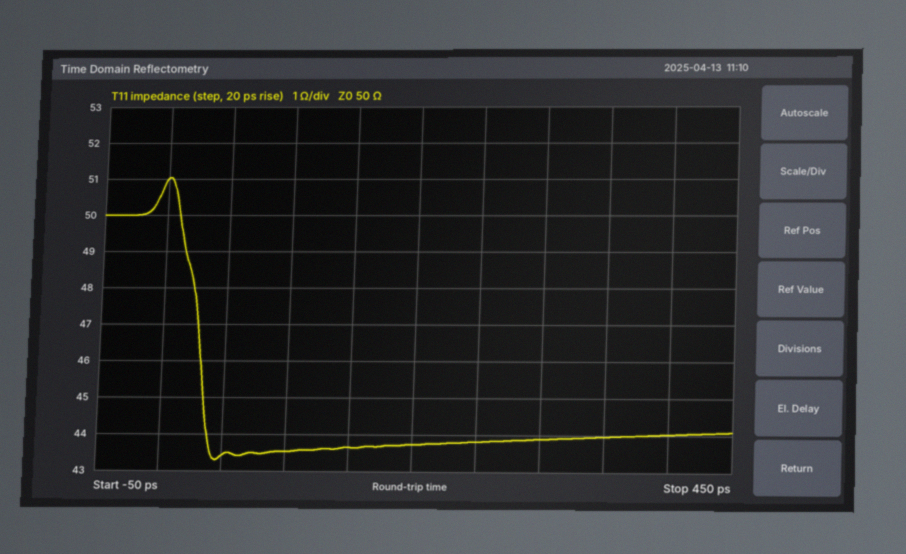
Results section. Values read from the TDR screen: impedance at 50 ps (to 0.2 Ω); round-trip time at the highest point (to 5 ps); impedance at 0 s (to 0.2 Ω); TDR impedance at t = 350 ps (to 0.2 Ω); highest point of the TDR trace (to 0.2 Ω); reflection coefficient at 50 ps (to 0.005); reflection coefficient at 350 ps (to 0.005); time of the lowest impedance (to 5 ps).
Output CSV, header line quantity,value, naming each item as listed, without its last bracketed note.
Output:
quantity,value
impedance at 50 ps,43.4 Ω
round-trip time at the highest point,0 ps
impedance at 0 s,51.0 Ω
TDR impedance at t = 350 ps,44.0 Ω
highest point of the TDR trace,51.0 Ω
reflection coefficient at 50 ps,-0.070
reflection coefficient at 350 ps,-0.065
time of the lowest impedance,45 ps
